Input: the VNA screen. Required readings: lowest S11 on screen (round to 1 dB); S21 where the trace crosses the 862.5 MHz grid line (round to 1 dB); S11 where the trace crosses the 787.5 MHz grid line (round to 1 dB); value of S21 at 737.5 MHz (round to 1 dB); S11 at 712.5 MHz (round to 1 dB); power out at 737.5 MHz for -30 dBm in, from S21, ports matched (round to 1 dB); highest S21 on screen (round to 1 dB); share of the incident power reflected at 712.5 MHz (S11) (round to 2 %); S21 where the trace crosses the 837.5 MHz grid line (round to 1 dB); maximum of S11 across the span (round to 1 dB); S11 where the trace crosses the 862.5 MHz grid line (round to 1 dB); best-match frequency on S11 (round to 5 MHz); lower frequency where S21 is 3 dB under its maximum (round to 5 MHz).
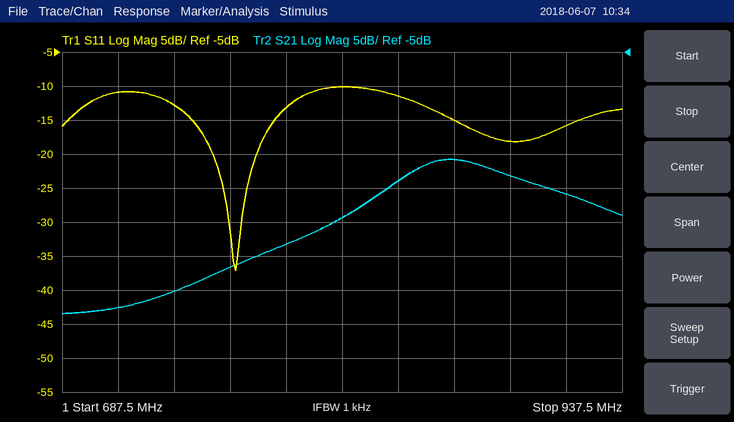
-37 dB
-21 dB
-13 dB
-40 dB
-11 dB
-70 dBm
-21 dB
8 %
-24 dB
-10 dB
-15 dB
765 MHz
840 MHz
